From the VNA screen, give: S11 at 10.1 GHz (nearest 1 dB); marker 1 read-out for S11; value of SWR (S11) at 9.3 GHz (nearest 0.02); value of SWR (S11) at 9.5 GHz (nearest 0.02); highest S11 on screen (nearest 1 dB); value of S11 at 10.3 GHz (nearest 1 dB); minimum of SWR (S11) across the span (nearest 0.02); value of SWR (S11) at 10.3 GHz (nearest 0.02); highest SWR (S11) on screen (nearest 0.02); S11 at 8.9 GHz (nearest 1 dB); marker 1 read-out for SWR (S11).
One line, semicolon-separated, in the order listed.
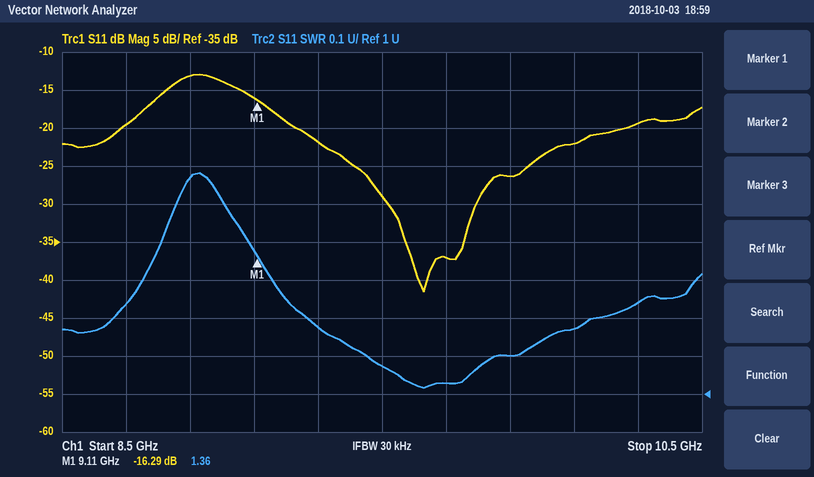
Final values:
-22 dB; -16.29 dB; 1.18; 1.08; -13 dB; -19 dB; 1.02; 1.24; 1.58; -13 dB; 1.36
